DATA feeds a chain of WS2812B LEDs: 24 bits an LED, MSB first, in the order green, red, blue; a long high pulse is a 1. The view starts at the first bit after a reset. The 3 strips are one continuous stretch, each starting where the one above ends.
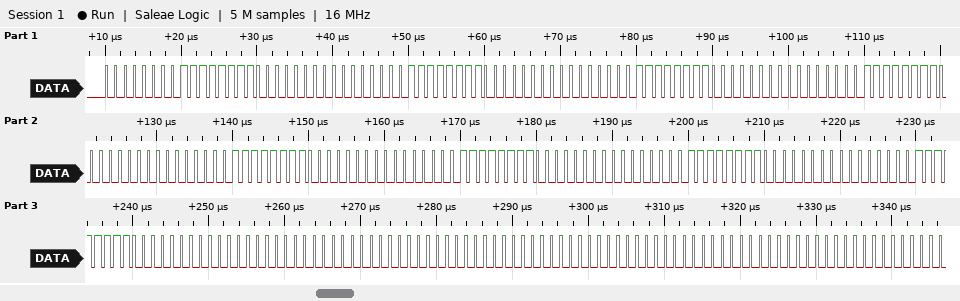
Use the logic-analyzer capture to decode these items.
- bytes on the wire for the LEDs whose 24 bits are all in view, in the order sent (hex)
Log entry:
00 FF 00 00 FF 00 00 FF 00 00 FF 00 00 FF 00 00 FF 00 00 FF 00 00 FF 00 00 00 00 00 00 00 00 00 00
